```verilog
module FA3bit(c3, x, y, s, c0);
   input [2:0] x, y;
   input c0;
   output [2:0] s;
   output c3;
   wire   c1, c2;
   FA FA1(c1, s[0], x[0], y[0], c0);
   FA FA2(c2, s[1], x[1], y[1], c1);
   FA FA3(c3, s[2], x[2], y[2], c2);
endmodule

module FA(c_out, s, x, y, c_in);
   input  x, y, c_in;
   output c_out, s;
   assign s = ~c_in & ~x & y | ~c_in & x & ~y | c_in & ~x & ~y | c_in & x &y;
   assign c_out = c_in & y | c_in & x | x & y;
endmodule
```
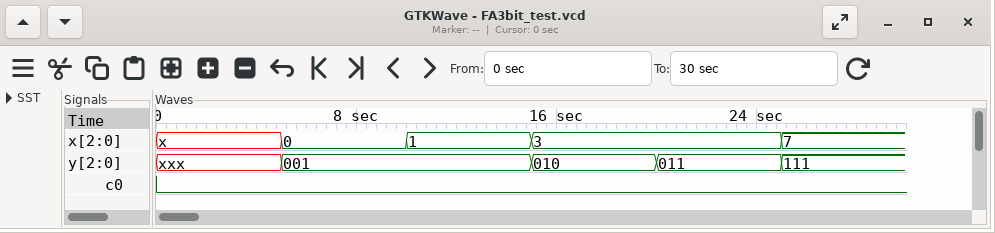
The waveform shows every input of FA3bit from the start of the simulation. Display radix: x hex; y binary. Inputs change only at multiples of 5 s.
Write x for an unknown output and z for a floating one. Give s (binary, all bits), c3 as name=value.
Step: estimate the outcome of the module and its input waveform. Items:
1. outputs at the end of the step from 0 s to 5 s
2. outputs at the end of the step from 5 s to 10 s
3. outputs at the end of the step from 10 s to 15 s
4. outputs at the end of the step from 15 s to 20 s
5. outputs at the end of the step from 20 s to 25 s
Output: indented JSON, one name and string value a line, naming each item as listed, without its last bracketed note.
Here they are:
{
  "outputs at the end of the step from 0 s to 5 s": "s=x, c3=x",
  "outputs at the end of the step from 5 s to 10 s": "s=001, c3=0",
  "outputs at the end of the step from 10 s to 15 s": "s=010, c3=0",
  "outputs at the end of the step from 15 s to 20 s": "s=101, c3=0",
  "outputs at the end of the step from 20 s to 25 s": "s=110, c3=0"
}
